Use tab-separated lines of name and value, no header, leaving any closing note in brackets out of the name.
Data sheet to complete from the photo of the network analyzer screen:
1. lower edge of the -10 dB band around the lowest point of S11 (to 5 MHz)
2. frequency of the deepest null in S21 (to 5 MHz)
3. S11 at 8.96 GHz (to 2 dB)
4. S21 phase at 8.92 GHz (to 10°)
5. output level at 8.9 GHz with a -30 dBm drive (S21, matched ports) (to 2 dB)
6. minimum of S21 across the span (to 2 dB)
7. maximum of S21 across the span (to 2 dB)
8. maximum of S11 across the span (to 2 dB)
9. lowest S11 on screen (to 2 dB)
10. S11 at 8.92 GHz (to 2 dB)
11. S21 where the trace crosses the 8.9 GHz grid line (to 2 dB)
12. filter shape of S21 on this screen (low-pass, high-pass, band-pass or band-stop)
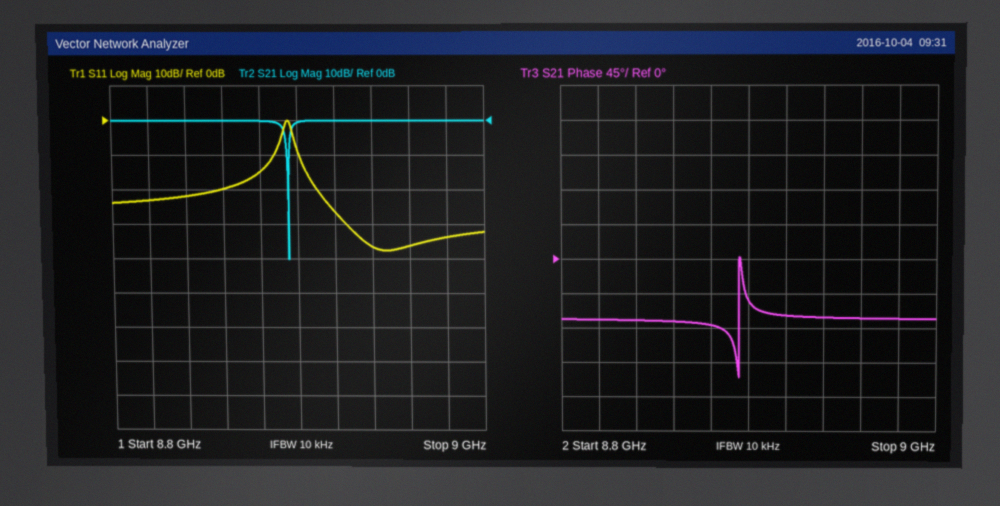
lower edge of the -10 dB band around the lowest point of S11	8.900 GHz
frequency of the deepest null in S21	8.895 GHz
S11 at 8.96 GHz	-36 dB
S21 phase at 8.92 GHz	-70°
output level at 8.9 GHz with a -30 dBm drive (S21, matched ports)	-30 dBm
minimum of S21 across the span	-40 dB
maximum of S21 across the span	0 dB
maximum of S11 across the span	0 dB
lowest S11 on screen	-38 dB
S11 at 8.92 GHz	-26 dB
S21 where the trace crosses the 8.9 GHz grid line	0 dB
filter shape of S21 on this screen	band-stop
